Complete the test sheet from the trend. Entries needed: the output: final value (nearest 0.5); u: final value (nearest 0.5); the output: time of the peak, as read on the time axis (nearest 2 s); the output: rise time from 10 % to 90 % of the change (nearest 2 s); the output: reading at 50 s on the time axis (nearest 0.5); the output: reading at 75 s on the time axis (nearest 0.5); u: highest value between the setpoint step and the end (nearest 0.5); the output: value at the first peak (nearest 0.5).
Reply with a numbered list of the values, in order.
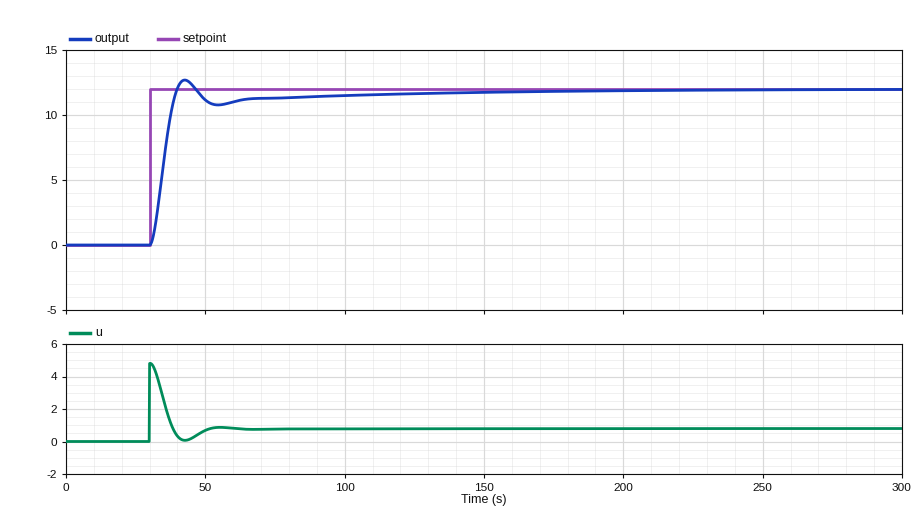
1. 12.0
2. 1.0
3. 42 s
4. 6 s
5. 11.0
6. 11.5
7. 5.0
8. 12.5
